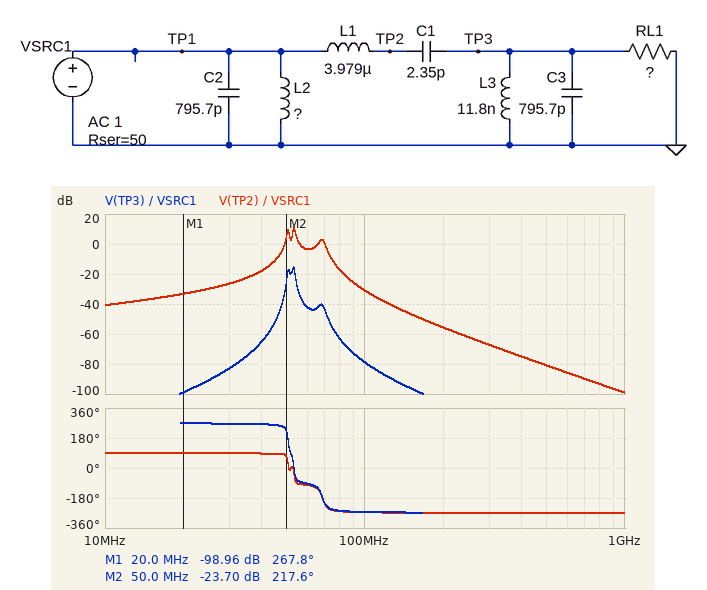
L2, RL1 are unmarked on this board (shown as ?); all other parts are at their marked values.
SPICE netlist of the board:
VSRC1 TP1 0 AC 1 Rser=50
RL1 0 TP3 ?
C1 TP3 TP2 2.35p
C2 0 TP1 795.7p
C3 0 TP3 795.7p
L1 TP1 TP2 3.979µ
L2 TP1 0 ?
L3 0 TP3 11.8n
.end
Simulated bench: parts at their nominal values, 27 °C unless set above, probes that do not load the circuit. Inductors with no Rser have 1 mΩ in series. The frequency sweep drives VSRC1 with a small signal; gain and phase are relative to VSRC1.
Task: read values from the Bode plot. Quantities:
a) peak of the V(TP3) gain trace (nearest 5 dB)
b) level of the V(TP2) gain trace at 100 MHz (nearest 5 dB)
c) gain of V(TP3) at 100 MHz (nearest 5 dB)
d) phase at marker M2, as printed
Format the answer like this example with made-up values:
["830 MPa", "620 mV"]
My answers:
["-15 dB", "-30 dB", "-80 dB", "217.6 deg"]
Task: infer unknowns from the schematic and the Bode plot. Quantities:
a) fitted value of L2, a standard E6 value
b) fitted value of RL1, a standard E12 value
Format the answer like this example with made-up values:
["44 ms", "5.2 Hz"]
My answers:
["6.8 nH", "100 Ω"]
